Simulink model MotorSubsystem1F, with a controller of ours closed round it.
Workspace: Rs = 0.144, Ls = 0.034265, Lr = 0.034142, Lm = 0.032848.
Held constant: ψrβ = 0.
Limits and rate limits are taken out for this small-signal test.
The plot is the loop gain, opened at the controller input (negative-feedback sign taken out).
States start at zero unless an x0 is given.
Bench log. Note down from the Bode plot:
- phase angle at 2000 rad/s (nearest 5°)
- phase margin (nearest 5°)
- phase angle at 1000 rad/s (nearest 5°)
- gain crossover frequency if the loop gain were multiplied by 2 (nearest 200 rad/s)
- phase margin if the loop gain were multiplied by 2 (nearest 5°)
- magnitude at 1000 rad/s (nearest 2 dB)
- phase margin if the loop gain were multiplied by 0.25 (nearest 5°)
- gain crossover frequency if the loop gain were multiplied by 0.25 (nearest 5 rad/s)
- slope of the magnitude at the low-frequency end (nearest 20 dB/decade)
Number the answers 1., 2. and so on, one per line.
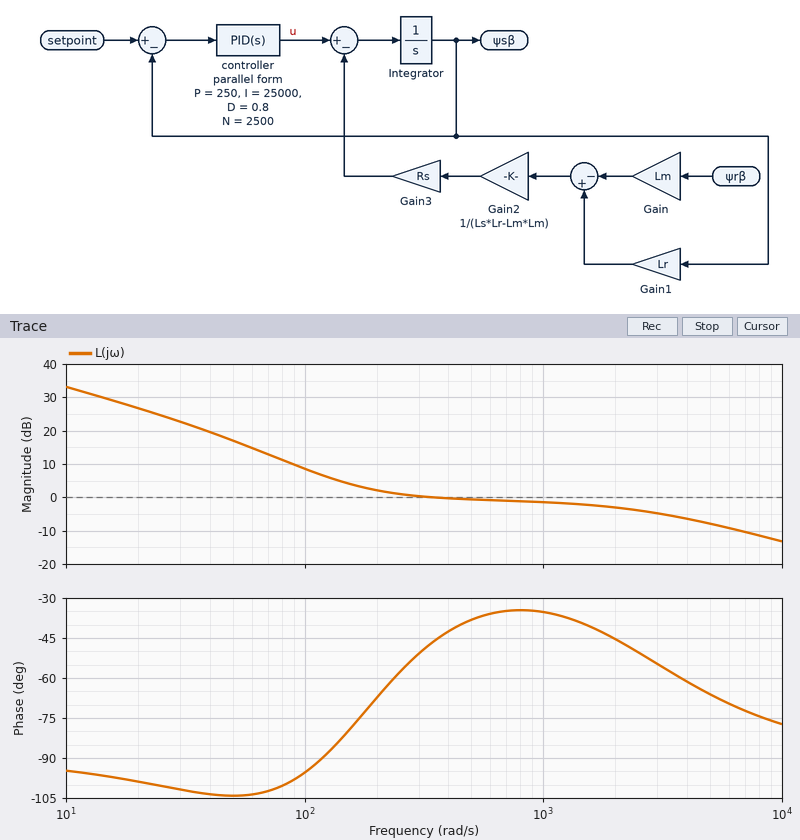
1. -45°
2. 135°
3. -35°
4. 3800 rad/s
5. 120°
6. -2 dB
7. 80°
8. 75 rad/s
9. -20 dB/decade
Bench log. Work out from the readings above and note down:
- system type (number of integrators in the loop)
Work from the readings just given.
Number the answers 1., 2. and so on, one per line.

1. 1
